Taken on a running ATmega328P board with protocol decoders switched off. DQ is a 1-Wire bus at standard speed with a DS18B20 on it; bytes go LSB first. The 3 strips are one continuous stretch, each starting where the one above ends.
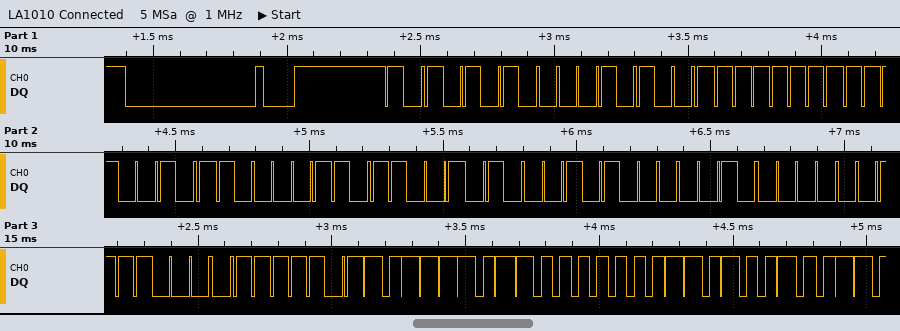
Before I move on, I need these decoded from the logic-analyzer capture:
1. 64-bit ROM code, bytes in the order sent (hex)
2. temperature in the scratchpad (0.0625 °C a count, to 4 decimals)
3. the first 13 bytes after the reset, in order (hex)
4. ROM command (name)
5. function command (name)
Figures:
28 FF A7 61 53 14 04 1C
27.8125 °C
55 28 FF A7 61 53 14 04 1C BE BD 01 4B
Match ROM
Read Scratchpad
